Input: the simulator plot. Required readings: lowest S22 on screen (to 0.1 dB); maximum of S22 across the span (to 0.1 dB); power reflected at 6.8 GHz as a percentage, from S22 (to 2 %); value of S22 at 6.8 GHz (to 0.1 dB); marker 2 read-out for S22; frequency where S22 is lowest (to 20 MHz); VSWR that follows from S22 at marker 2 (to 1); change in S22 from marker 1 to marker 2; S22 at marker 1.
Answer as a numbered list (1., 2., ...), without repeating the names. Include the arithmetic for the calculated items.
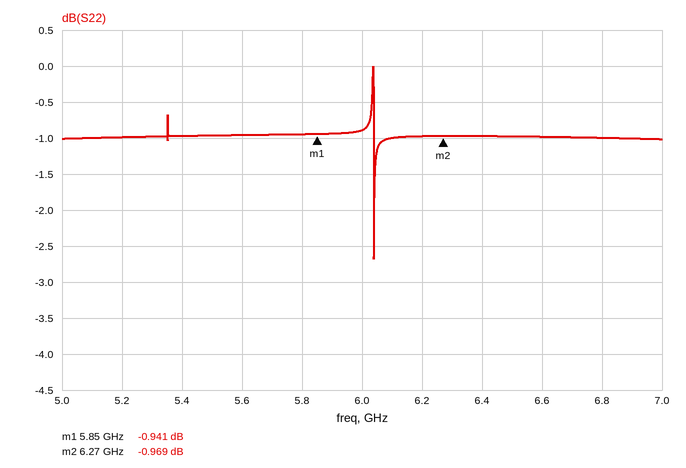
1. -2.7 dB
2. 0.0 dB
3. 10^(-1/10) ≈ 79.4 %, so 80 % to the nearest 2 %
4. -1.0 dB
5. -0.969 dB
6. 6.04 GHz
7. (1 + 0.8944)/(1 − 0.8944) ≈ 18
8. -0.969 − (-0.941) = -0.028 dB
9. -0.941 dB
